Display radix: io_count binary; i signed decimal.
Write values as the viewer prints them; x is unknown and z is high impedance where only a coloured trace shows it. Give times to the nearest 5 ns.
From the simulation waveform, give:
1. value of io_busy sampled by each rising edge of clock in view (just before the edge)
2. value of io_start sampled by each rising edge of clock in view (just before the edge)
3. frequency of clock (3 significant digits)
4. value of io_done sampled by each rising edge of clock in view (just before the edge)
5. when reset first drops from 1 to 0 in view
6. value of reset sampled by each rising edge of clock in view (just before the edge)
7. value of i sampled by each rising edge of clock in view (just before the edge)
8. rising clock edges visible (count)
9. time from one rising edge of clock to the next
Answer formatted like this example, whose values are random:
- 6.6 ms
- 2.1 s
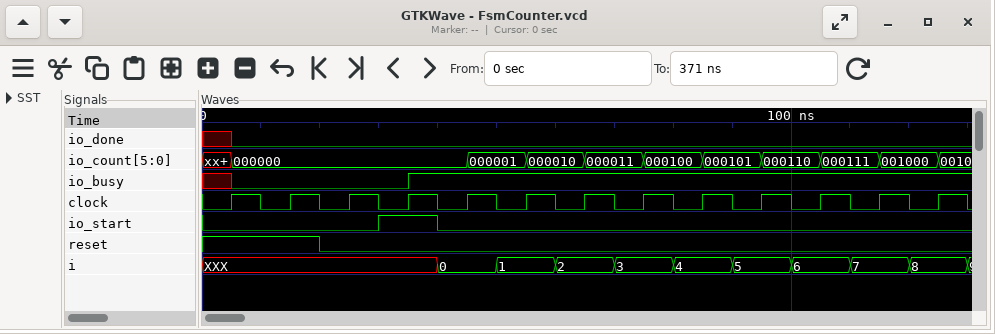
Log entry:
- x 0 0 0 1 1 1 1 1 1 1 1 1
- 0 0 0 1 0 0 0 0 0 0 0 0 0
- 100 MHz
- x 0 0 0 0 0 0 0 0 0 0 0 0
- 20 ns
- 1 1 0 0 0 0 0 0 0 0 0 0 0
- XXX, XXX, XXX, XXX, 0, 1, 2, 3, 4, 5, 6, 7, 8
- 13
- 10 ns
